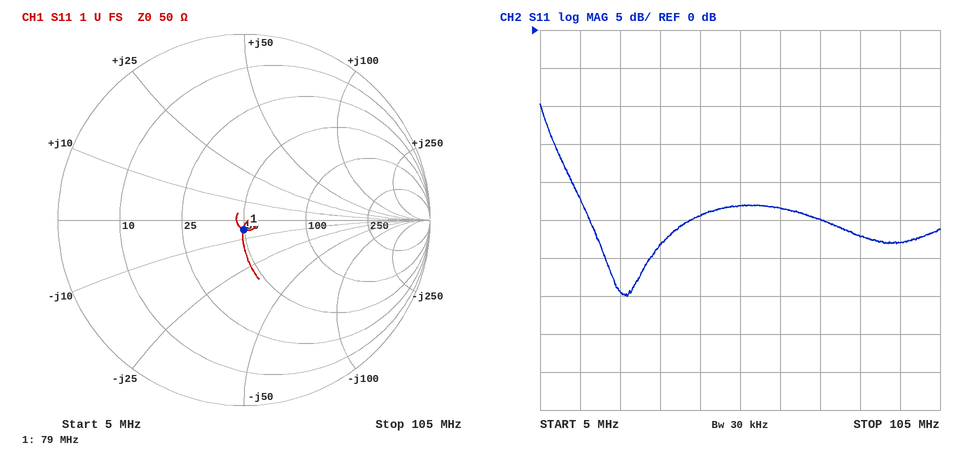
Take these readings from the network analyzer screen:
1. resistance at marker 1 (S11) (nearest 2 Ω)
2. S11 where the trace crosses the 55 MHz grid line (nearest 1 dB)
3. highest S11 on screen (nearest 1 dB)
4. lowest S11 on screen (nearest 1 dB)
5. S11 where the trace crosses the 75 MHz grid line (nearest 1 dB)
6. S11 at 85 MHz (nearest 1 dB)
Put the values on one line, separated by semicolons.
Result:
50 Ω; -23 dB; -10 dB; -35 dB; -25 dB; -27 dB
